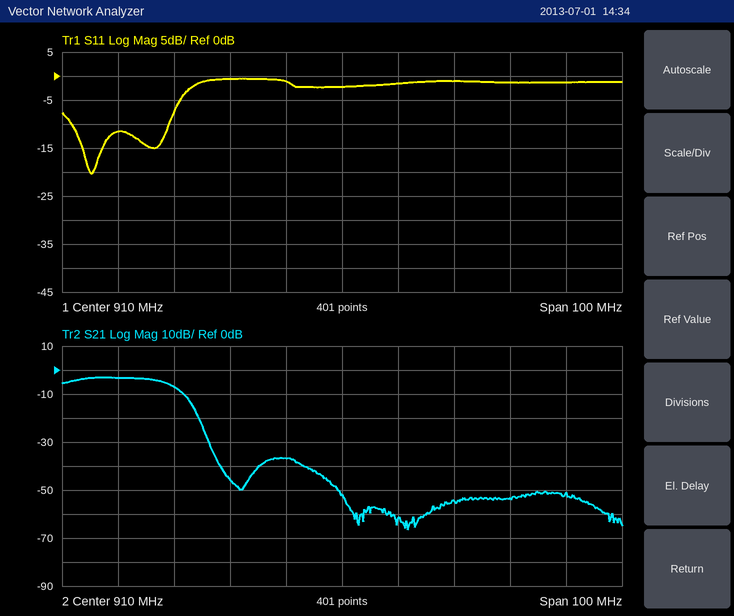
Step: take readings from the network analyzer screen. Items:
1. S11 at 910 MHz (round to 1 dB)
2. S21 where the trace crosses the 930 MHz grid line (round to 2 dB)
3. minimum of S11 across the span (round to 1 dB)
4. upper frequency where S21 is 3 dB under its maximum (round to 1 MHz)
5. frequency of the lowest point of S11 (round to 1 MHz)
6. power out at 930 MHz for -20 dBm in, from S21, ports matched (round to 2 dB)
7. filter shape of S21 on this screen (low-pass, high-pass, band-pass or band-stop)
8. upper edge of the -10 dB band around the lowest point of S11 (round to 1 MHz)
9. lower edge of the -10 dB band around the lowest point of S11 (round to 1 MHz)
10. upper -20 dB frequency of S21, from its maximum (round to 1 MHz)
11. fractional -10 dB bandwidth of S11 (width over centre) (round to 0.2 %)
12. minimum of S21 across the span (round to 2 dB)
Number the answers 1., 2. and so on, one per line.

1. -2 dB
2. -54 dB
3. -20 dB
4. 879 MHz
5. 865 MHz
6. -74 dBm
7. low-pass
8. 879 MHz
9. 862 MHz
10. 885 MHz
11. 2.0 %
12. -66 dB
